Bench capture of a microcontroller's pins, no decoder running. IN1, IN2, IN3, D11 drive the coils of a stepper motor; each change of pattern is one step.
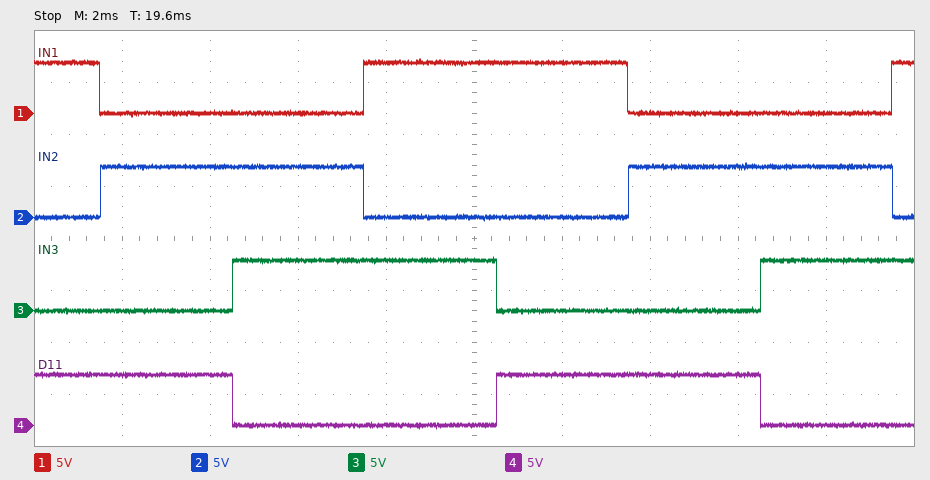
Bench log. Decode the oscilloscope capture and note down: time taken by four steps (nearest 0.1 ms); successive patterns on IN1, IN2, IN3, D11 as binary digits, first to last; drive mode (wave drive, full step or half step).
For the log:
12.0 ms
1001 0101 0110 1010 1001 0101 0110 1010
full step
